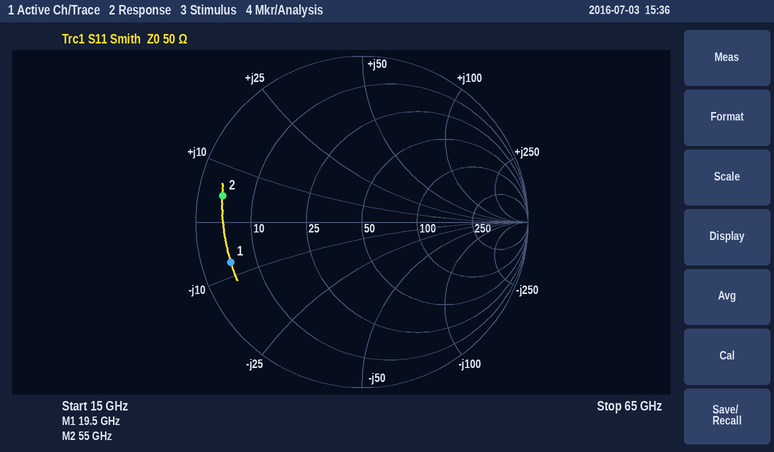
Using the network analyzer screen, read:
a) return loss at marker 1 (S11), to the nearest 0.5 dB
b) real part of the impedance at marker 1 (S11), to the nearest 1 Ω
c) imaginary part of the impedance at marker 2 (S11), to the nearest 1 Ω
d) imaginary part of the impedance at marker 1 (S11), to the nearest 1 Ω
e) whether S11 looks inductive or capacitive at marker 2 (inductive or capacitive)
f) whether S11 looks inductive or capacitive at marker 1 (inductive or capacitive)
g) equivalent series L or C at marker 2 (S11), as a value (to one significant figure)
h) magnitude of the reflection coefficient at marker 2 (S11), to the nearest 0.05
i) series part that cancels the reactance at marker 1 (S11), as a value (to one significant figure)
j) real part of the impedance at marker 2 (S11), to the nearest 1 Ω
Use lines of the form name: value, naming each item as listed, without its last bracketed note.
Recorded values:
return loss at marker 1 (S11), to the nearest 0.5 dB: 1.5 dB
real part of the impedance at marker 1 (S11), to the nearest 1 Ω: 5 Ω
imaginary part of the impedance at marker 2 (S11), to the nearest 1 Ω: +5 Ω
imaginary part of the impedance at marker 1 (S11), to the nearest 1 Ω: -7 Ω
whether S11 looks inductive or capacitive at marker 2: inductive
whether S11 looks inductive or capacitive at marker 1: capacitive
equivalent series L or C at marker 2 (S11), as a value: 10 pH
magnitude of the reflection coefficient at marker 2 (S11), to the nearest 0.05: 0.85
series part that cancels the reactance at marker 1 (S11), as a value: 60 pH
real part of the impedance at marker 2 (S11), to the nearest 1 Ω: 4 Ω
